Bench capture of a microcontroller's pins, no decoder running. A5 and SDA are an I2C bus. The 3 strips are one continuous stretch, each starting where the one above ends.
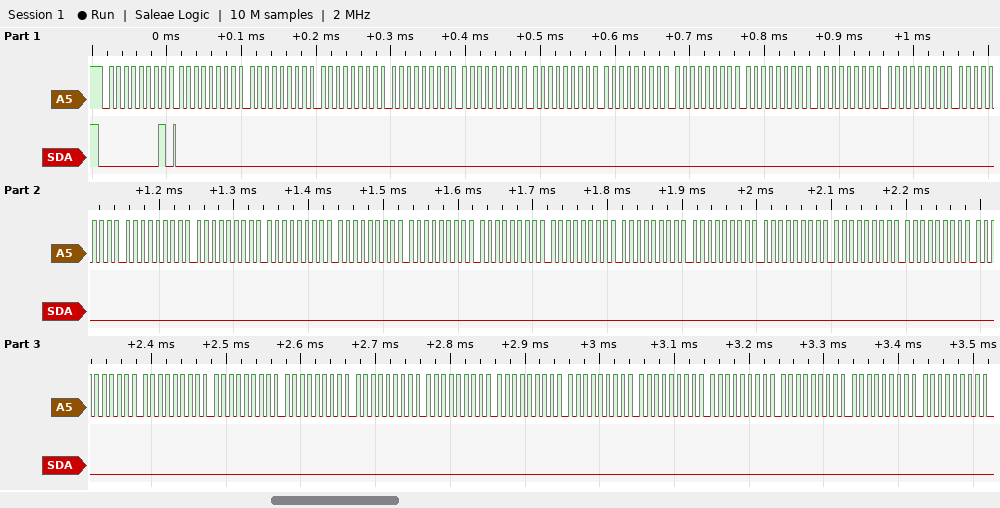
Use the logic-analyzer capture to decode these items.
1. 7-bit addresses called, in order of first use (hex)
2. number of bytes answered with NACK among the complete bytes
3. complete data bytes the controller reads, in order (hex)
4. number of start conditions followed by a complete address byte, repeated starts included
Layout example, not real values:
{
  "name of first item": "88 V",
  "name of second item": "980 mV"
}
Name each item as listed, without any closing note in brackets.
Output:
{
  "7-bit addresses called, in order of first use": "0x00",
  "number of bytes answered with NACK among the complete bytes": "0",
  "complete data bytes the controller reads, in order": "00 00 00 00 00 00 00 00 00 00 00 00 00 00 00 00 00 00 00 00 00 00 00 00 00 00 00 00 00 00 00 00 00 00 00 00 00",
  "number of start conditions followed by a complete address byte, repeated starts included": "1"
}
